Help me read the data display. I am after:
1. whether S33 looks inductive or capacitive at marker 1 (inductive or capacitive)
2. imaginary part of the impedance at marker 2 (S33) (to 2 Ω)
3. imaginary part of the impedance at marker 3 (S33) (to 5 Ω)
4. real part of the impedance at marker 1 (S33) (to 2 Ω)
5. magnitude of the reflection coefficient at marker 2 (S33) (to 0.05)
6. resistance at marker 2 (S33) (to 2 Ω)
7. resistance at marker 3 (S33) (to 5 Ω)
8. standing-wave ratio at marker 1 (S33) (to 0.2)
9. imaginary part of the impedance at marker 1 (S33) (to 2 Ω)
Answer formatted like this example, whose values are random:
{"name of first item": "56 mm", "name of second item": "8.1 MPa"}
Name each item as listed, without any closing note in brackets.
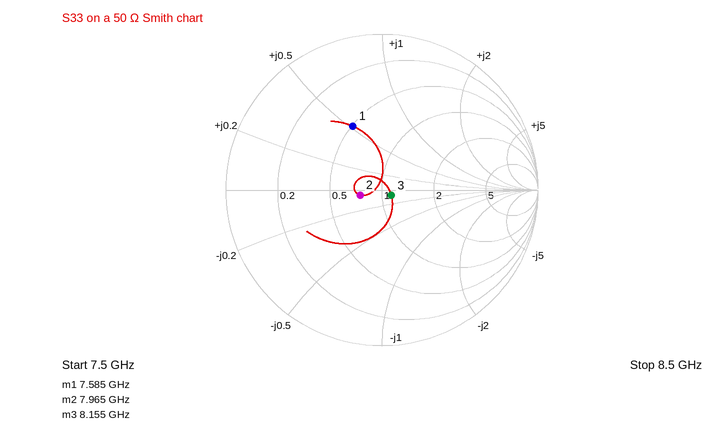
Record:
{"whether S33 looks inductive or capacitive at marker 1": "inductive", "imaginary part of the impedance at marker 2 (S33)": "-2 Ω", "imaginary part of the impedance at marker 3 (S33)": "-5 Ω", "real part of the impedance at marker 1 (S33)": "26 Ω", "magnitude of the reflection coefficient at marker 2 (S33)": "0.15", "resistance at marker 2 (S33)": "38 Ω", "resistance at marker 3 (S33)": "55 Ω", "standing-wave ratio at marker 1 (S33)": "2.6", "imaginary part of the impedance at marker 1 (S33)": "+26 Ω"}
